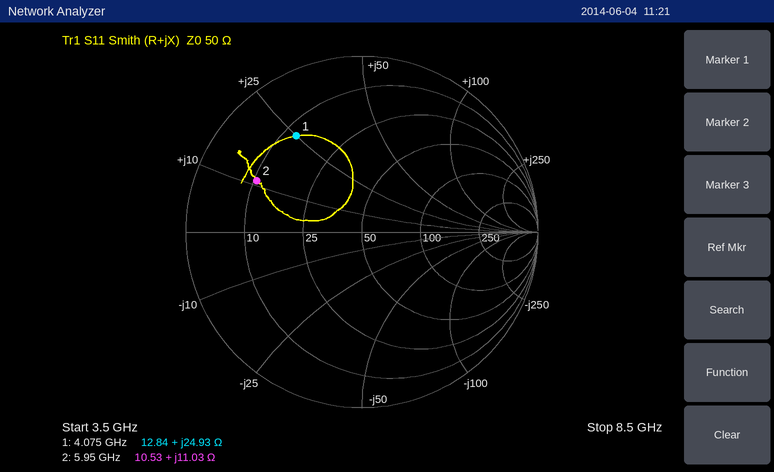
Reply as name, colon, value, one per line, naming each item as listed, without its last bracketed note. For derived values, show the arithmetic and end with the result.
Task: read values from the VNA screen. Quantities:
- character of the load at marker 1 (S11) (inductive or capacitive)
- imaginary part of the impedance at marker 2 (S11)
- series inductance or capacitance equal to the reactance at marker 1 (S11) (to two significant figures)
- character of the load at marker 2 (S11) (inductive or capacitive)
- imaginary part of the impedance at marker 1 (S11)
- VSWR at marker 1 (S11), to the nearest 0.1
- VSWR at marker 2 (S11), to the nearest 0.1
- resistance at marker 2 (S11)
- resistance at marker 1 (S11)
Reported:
character of the load at marker 1 (S11): inductive
imaginary part of the impedance at marker 2: +11.03 Ω
series inductance or capacitance equal to the reactance at marker 1 (S11): L = 24.93 Ω/(2π × 4.075 GHz) ≈ 974 pH, so 970 pH to two significant figures
character of the load at marker 2 (S11): inductive
imaginary part of the impedance at marker 1: +24.93 Ω
VSWR at marker 1 (S11), to the nearest 0.1: 4.9
VSWR at marker 2 (S11), to the nearest 0.1: 5.0
resistance at marker 2: 10.53 Ω
resistance at marker 1: 12.84 Ω
